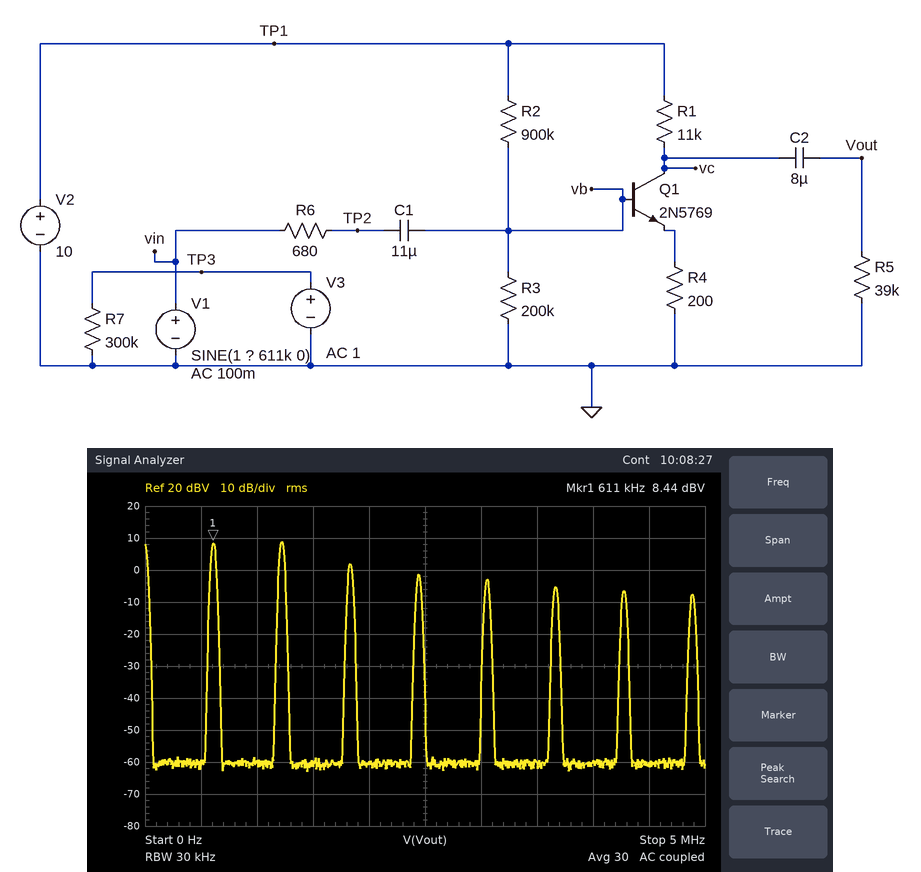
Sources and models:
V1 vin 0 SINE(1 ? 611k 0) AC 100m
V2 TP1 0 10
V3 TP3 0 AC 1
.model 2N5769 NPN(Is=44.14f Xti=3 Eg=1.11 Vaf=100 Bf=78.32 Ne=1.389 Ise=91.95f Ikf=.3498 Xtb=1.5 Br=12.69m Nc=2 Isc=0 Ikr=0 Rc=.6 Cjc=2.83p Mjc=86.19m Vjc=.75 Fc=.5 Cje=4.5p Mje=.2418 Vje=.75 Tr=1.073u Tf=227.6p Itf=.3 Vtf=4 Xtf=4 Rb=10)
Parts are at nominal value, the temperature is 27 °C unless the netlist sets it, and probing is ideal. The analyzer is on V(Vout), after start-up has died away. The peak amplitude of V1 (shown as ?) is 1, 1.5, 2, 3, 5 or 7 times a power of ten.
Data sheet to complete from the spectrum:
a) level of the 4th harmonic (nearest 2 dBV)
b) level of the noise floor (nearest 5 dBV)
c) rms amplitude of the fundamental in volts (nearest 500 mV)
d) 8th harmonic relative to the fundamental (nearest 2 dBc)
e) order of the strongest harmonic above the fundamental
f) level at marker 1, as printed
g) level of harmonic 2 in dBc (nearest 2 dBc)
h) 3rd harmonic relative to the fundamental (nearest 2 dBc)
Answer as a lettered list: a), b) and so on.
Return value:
a) -2 dBV
b) -60 dBV
c) 2.5 V
d) -16 dBc
e) 2
f) 8.44 dBV
g) 0 dBc
h) -6 dBc
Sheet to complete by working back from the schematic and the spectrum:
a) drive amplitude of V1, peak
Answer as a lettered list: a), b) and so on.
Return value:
a) 70 V
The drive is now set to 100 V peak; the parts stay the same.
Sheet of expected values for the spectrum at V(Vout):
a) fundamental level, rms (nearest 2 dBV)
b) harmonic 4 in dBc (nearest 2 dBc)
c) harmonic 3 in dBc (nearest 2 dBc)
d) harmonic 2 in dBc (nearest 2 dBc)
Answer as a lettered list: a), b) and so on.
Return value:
a) 14 dBV
b) -12 dBc
c) -12 dBc
d) -2 dBc
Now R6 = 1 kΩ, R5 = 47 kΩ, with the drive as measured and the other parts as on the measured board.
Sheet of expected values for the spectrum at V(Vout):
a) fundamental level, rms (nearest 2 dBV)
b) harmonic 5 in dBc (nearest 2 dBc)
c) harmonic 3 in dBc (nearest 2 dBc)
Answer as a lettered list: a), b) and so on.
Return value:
a) 6 dBV
b) -10 dBc
c) -4 dBc
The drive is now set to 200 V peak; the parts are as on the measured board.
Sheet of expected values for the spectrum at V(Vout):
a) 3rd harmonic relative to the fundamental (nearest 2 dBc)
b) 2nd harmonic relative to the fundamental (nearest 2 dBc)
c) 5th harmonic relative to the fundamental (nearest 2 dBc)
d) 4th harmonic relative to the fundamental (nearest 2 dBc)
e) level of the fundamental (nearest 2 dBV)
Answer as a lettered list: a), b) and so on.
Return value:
a) -20 dBc
b) -4 dBc
c) -26 dBc
d) -16 dBc
e) 22 dBV
